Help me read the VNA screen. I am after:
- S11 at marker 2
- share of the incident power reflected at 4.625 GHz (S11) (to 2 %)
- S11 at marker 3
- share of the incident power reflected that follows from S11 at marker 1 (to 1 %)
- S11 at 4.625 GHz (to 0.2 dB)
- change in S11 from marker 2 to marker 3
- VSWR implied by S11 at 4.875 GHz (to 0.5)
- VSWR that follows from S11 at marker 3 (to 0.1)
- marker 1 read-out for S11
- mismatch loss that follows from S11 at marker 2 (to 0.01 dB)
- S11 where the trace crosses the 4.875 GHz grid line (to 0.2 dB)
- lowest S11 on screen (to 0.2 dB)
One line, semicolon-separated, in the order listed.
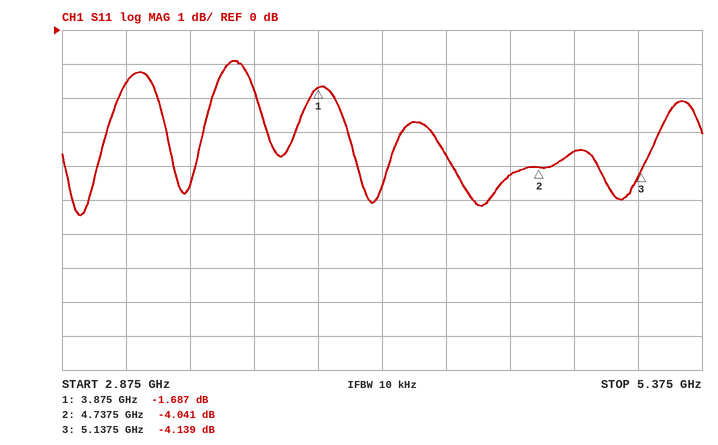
-4.041 dB; 38 %; -4.139 dB; 68 %; -4.2 dB; -0.098 dB; 5.0; 4.3; -1.687 dB; 2.18 dB; -3.6 dB; -5.4 dB
